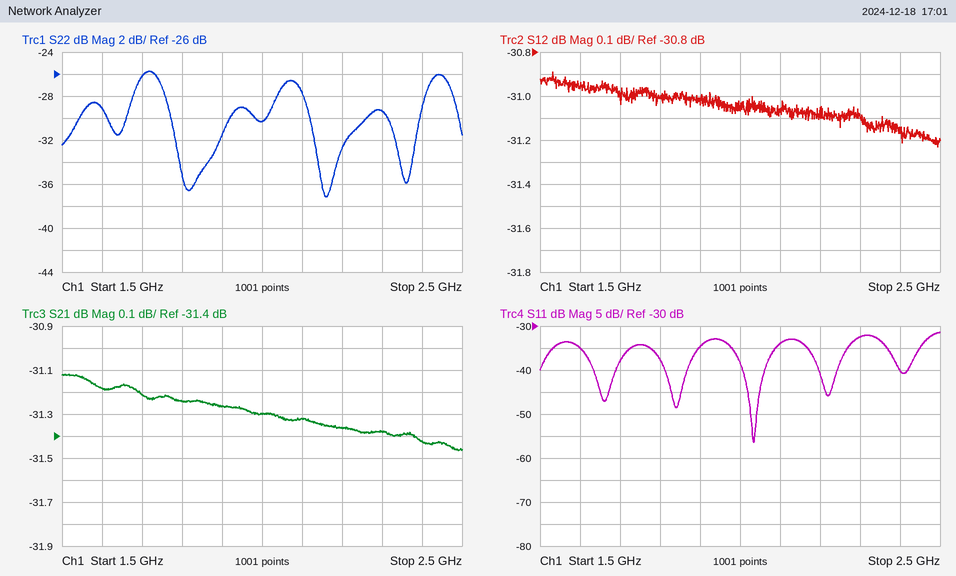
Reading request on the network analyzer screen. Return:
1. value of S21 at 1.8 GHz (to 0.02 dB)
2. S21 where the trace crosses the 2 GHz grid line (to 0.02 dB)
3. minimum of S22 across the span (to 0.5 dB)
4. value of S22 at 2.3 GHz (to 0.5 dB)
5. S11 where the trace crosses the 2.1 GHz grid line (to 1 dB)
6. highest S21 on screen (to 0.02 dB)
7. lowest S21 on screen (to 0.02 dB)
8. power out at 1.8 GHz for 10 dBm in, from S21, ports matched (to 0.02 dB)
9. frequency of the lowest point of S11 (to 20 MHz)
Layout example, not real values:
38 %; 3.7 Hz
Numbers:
-31.24 dB; -31.30 dB; -37.0 dB; -29.5 dB; -34 dB; -31.12 dB; -31.46 dB; -21.24 dBm; 2.04 GHz
